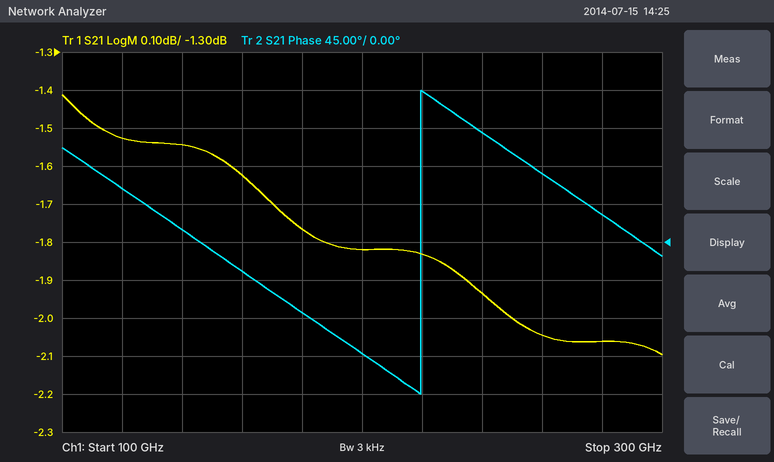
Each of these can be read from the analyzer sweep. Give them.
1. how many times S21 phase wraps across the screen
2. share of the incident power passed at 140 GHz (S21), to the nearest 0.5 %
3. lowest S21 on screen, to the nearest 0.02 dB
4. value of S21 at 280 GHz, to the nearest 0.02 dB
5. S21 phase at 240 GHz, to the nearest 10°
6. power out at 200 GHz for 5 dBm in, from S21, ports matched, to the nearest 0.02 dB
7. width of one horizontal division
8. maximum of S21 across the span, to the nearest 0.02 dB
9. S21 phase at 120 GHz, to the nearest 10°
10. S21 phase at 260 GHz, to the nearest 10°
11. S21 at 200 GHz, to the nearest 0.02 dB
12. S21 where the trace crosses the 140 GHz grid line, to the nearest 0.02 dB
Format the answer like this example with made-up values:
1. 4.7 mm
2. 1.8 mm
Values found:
1. 1
2. 70.0 %
3. -2.10 dB
4. -2.06 dB
5. 130°
6. 3.18 dBm
7. 20 GHz
8. -1.42 dB
9. 60°
10. 80°
11. -1.82 dB
12. -1.54 dB
